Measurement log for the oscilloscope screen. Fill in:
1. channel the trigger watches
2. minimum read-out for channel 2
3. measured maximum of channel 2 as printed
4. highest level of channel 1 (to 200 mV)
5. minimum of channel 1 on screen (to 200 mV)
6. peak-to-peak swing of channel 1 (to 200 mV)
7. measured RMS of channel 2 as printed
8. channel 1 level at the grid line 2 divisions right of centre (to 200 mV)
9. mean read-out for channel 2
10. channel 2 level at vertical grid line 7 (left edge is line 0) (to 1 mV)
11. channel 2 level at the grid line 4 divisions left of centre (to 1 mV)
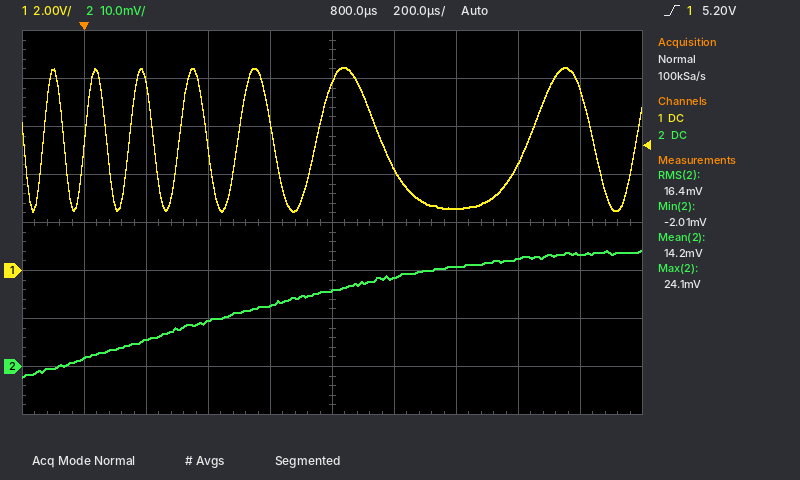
channel 1
-2.01 mV
24.1 mV
8.4 V
2.4 V
6.0 V
16.4 mV
2.6 V
14.2 mV
21 mV
2 mV
